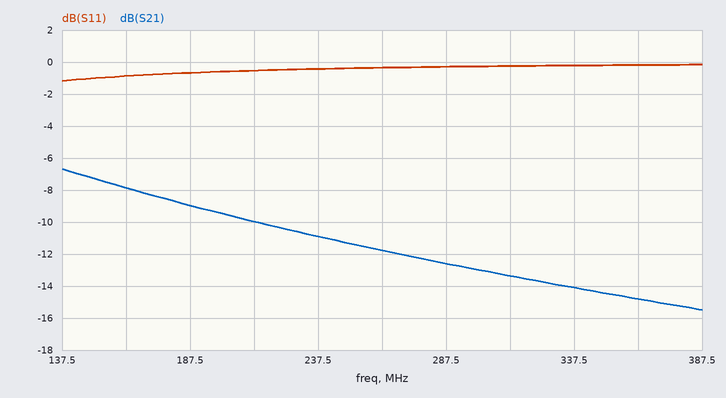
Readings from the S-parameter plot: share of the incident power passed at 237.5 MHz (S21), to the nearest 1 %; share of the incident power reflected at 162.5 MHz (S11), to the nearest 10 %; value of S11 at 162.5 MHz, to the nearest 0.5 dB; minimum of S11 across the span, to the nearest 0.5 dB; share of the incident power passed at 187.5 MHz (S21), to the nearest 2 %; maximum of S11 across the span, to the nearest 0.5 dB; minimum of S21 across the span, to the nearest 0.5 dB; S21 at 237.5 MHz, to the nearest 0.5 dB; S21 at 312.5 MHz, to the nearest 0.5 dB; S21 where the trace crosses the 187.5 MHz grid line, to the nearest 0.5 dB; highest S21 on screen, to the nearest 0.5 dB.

8 %
80 %
-1.0 dB
-1.0 dB
12 %
0.0 dB
-15.5 dB
-11.0 dB
-13.5 dB
-9.0 dB
-6.5 dB
